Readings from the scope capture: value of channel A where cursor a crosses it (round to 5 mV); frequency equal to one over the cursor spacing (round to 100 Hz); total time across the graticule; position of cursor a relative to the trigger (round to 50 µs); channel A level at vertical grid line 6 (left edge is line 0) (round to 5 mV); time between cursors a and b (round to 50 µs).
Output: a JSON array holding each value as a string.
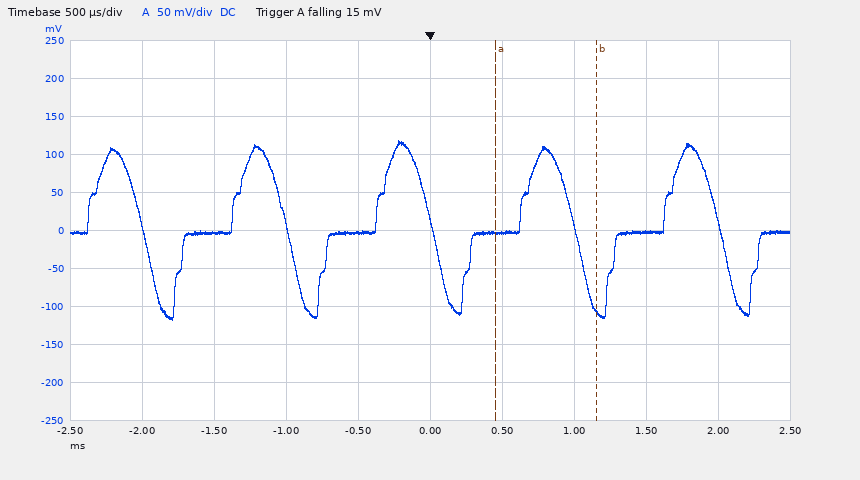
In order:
["-5 mV", "1.4 kHz", "5 ms", "+450 µs", "-5 mV", "700 µs"]
